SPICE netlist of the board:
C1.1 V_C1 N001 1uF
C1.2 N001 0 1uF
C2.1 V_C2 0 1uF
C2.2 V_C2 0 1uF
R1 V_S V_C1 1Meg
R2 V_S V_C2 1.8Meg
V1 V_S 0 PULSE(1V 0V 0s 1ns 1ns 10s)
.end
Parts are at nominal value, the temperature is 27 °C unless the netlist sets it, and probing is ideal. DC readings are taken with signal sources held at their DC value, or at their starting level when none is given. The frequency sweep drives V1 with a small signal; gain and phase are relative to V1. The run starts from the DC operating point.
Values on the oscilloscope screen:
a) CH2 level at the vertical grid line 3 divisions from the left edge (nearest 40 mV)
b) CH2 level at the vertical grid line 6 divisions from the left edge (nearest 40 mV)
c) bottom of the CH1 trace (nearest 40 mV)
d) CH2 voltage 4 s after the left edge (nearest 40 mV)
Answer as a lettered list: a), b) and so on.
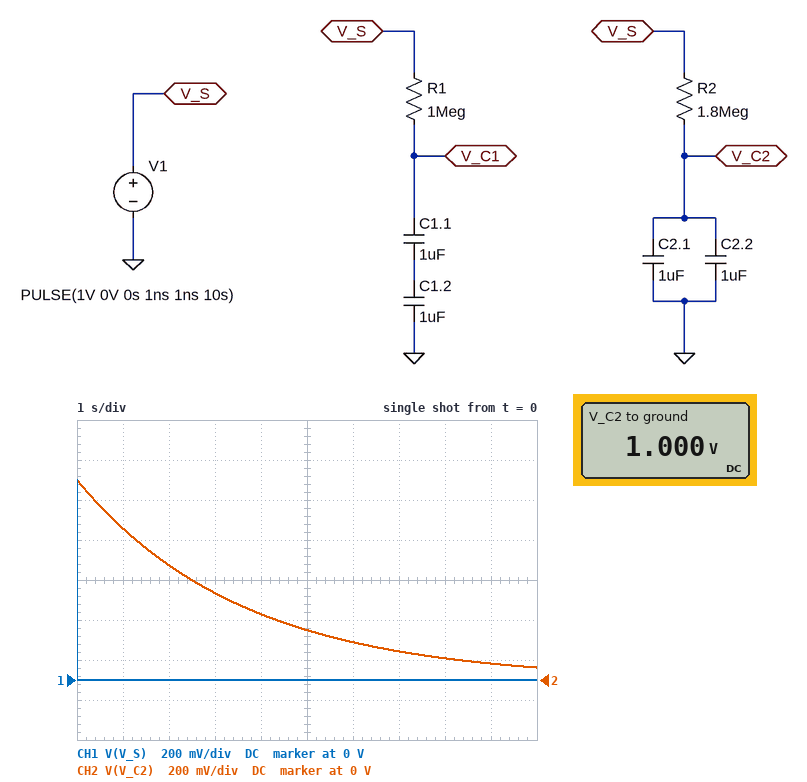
a) 440 mV
b) 200 mV
c) 0 V
d) 320 mV
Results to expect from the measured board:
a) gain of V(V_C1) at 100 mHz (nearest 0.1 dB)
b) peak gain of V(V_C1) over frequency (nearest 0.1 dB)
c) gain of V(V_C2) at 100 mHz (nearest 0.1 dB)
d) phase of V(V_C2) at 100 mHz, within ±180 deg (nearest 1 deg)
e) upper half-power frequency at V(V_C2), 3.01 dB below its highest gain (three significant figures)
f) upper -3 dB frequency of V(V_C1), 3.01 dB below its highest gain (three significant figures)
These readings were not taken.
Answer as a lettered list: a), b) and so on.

a) -0.4 dB
b) 0 dB
c) -7.9 dB
d) -66 deg
e) 44.2 mHz
f) 318 mHz
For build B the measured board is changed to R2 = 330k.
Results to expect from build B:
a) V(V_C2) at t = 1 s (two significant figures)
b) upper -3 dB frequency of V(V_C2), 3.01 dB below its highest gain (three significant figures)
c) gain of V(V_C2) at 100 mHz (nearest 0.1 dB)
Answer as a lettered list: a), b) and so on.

a) 220 mV
b) 241 mHz
c) -0.7 dB
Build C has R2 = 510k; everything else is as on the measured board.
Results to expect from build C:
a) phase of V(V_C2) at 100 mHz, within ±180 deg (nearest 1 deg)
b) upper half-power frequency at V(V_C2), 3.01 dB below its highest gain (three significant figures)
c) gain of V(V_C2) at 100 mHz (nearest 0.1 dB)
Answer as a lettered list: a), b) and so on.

a) -33 deg
b) 156 mHz
c) -1.5 dB
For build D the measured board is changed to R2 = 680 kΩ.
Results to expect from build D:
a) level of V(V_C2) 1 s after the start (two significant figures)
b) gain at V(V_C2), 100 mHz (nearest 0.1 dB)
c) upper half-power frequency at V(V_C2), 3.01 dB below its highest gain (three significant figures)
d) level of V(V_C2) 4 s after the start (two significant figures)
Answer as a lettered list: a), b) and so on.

a) 480 mV
b) -2.4 dB
c) 117 mHz
d) 53 mV
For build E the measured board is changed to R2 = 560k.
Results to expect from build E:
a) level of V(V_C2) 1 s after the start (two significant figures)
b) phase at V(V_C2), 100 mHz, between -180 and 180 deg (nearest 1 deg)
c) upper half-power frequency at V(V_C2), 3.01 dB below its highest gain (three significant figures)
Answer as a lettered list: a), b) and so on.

a) 410 mV
b) -35 deg
c) 142 mHz
